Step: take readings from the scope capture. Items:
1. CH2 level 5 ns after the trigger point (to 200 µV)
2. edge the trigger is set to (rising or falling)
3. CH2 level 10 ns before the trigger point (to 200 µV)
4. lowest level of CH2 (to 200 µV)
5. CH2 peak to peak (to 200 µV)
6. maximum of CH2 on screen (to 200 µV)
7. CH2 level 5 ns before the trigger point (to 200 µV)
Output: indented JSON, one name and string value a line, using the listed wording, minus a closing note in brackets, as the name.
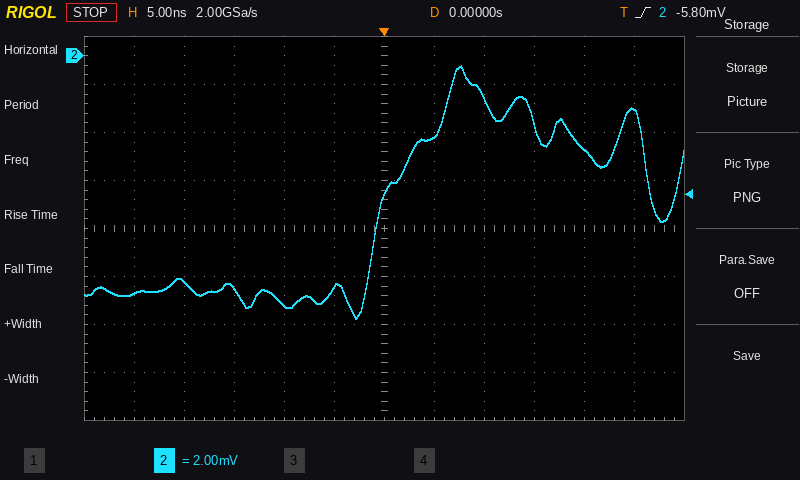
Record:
{
  "CH2 level 5 ns after the trigger point": "-3.4 mV",
  "edge the trigger is set to": "rising",
  "CH2 level 10 ns before the trigger point": "-10.4 mV",
  "lowest level of CH2": "-11.0 mV",
  "CH2 peak to peak": "10.6 mV",
  "maximum of CH2 on screen": "-400 µV",
  "CH2 level 5 ns before the trigger point": "-9.6 mV"
}
